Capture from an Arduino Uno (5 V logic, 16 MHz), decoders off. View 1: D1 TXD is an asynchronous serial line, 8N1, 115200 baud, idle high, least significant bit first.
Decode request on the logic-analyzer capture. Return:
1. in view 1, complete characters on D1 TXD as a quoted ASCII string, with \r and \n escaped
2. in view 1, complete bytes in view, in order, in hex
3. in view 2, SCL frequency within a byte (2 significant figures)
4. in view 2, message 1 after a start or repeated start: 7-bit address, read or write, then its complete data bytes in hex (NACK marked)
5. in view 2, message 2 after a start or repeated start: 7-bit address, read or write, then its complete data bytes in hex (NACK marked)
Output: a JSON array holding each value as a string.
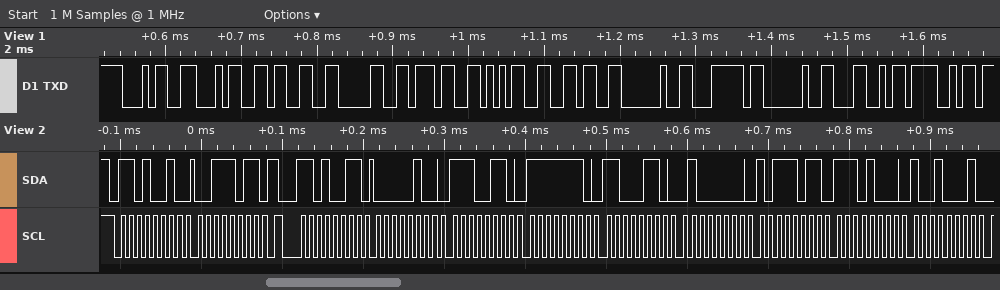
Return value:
["\"4430756 | LO\"", "34 34 33 30 37 35 36 20 7C 20 4C 4F", "100 kHz", "0x69 write: 3B", "0x69 read: 04 E6 FE C6 40 BB E8 91"]
